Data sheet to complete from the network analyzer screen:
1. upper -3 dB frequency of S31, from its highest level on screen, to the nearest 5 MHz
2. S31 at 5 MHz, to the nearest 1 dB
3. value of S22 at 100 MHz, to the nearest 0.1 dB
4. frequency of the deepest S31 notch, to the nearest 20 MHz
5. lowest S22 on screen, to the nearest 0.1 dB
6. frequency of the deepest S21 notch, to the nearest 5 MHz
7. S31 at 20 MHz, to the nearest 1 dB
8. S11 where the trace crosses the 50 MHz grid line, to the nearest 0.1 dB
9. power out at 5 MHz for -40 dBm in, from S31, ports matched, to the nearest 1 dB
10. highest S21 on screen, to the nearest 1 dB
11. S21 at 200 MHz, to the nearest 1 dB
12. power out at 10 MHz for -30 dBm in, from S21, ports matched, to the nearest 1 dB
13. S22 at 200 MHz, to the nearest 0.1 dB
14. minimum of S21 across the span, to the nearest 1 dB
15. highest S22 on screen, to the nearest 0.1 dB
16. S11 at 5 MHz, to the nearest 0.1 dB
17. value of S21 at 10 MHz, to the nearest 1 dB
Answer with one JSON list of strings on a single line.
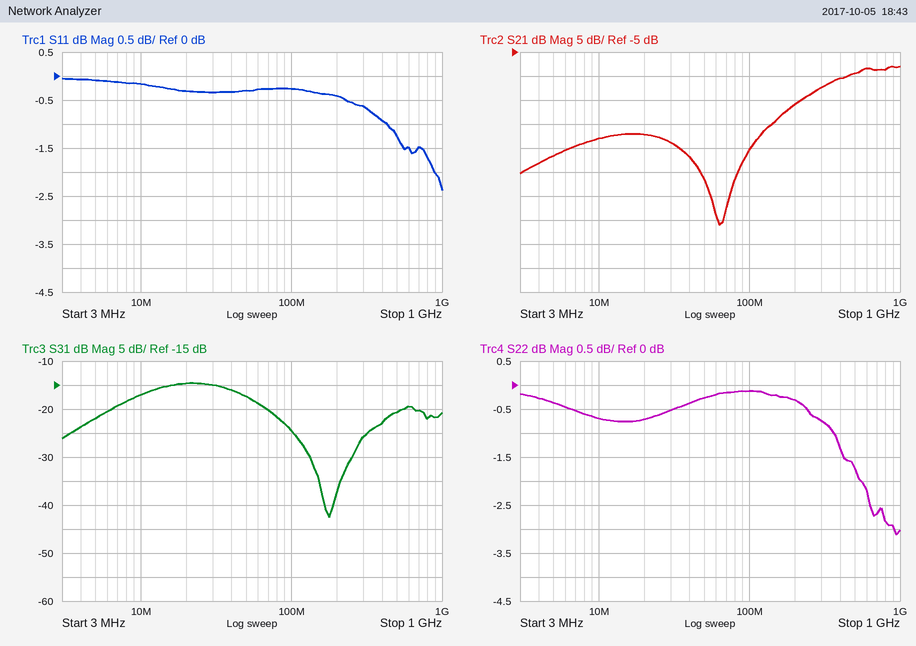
["50 MHz", "-22 dB", "-0.1 dB", "180 MHz", "-3.1 dB", "65 MHz", "-15 dB", "-0.3 dB", "-62 dBm", "-8 dB", "-16 dB", "-53 dBm", "-0.3 dB", "-41 dB", "-0.1 dB", "-0.1 dB", "-23 dB"]
